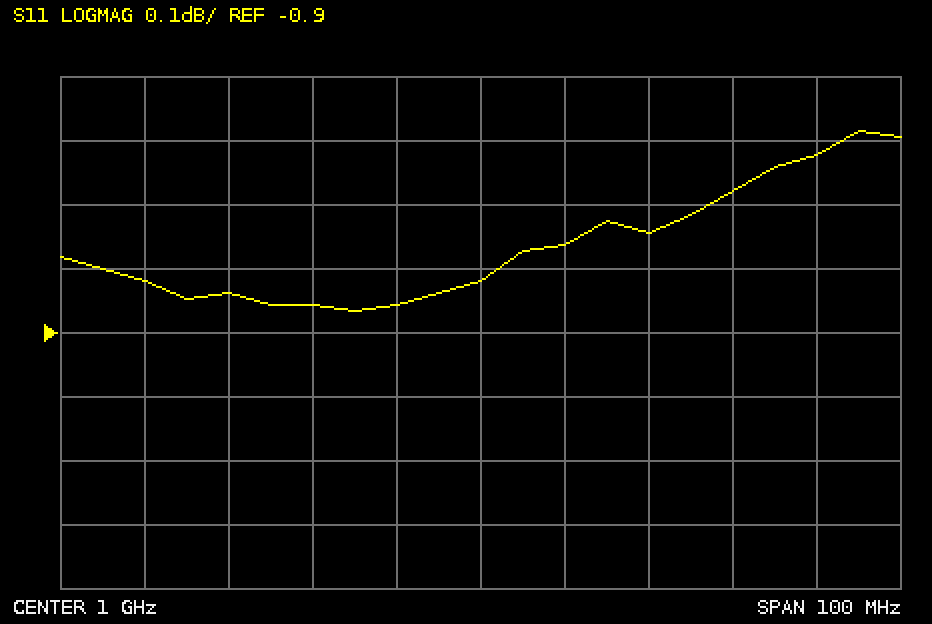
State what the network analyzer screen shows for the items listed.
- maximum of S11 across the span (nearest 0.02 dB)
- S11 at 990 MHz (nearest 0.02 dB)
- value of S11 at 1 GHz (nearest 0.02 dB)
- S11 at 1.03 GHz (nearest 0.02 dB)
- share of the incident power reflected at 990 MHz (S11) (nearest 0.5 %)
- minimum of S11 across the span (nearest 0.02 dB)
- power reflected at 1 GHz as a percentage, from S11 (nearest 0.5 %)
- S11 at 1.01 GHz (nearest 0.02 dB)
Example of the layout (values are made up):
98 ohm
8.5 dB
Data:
-0.58 dB
-0.86 dB
-0.82 dB
-0.68 dB
82.0 %
-0.86 dB
83.0 %
-0.76 dB
